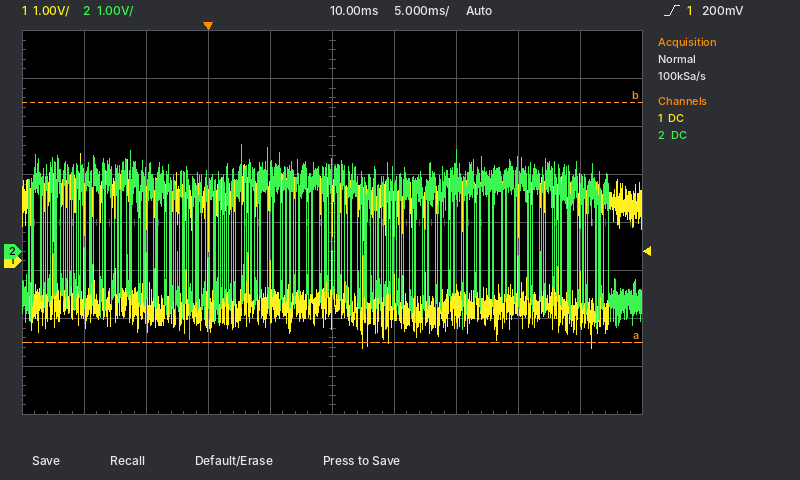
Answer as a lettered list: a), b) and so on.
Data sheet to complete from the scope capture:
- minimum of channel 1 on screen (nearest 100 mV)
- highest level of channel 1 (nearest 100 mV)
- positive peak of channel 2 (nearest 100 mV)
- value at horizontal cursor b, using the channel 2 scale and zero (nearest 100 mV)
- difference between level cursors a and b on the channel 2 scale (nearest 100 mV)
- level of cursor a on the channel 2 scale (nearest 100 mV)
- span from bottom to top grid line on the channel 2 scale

a) -1.8 V
b) 2.2 V
c) 2.2 V
d) 3.1 V
e) 5.0 V
f) -1.9 V
g) 8 V
